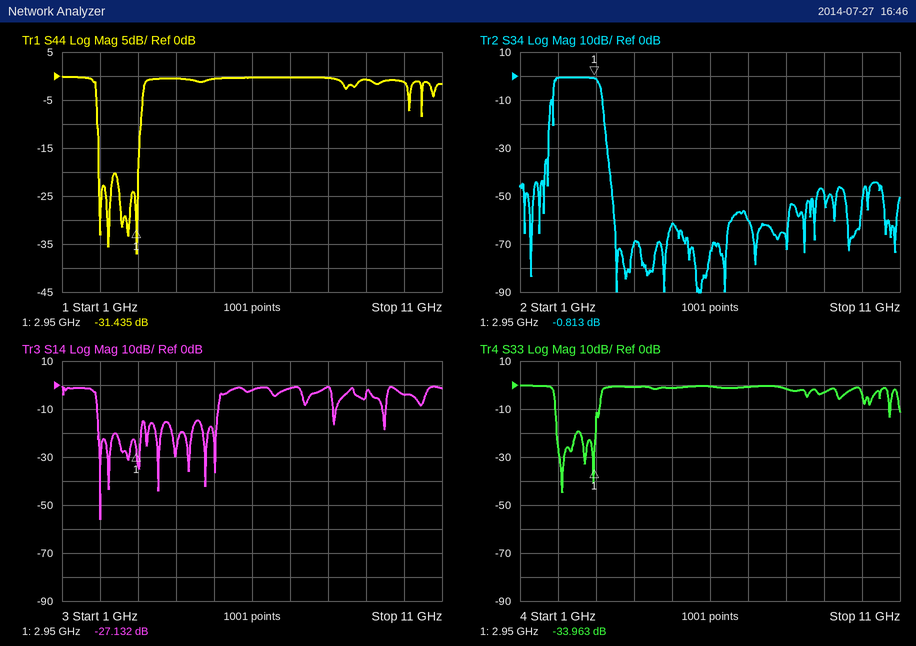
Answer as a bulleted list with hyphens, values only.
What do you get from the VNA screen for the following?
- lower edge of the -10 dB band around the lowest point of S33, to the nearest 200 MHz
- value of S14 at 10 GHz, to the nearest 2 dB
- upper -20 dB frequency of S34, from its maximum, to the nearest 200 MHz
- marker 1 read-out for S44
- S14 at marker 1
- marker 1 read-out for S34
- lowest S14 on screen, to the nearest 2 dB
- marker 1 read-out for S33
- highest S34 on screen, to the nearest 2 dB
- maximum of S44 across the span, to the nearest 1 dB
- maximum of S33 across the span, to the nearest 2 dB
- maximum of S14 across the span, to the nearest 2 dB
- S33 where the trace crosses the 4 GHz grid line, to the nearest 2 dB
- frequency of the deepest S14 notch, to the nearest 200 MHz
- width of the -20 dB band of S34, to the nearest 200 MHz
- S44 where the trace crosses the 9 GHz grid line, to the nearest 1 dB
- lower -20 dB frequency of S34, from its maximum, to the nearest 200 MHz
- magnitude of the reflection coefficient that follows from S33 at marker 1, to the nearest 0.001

- 2.0 GHz
- -4 dB
- 3.2 GHz
- -31.435 dB
- -27.132 dB
- -0.813 dB
- -56 dB
- -33.963 dB
- 0 dB
- 0 dB
- 0 dB
- 0 dB
- 0 dB
- 2.0 GHz
- 1.4 GHz
- -1 dB
- 1.8 GHz
- 0.020
